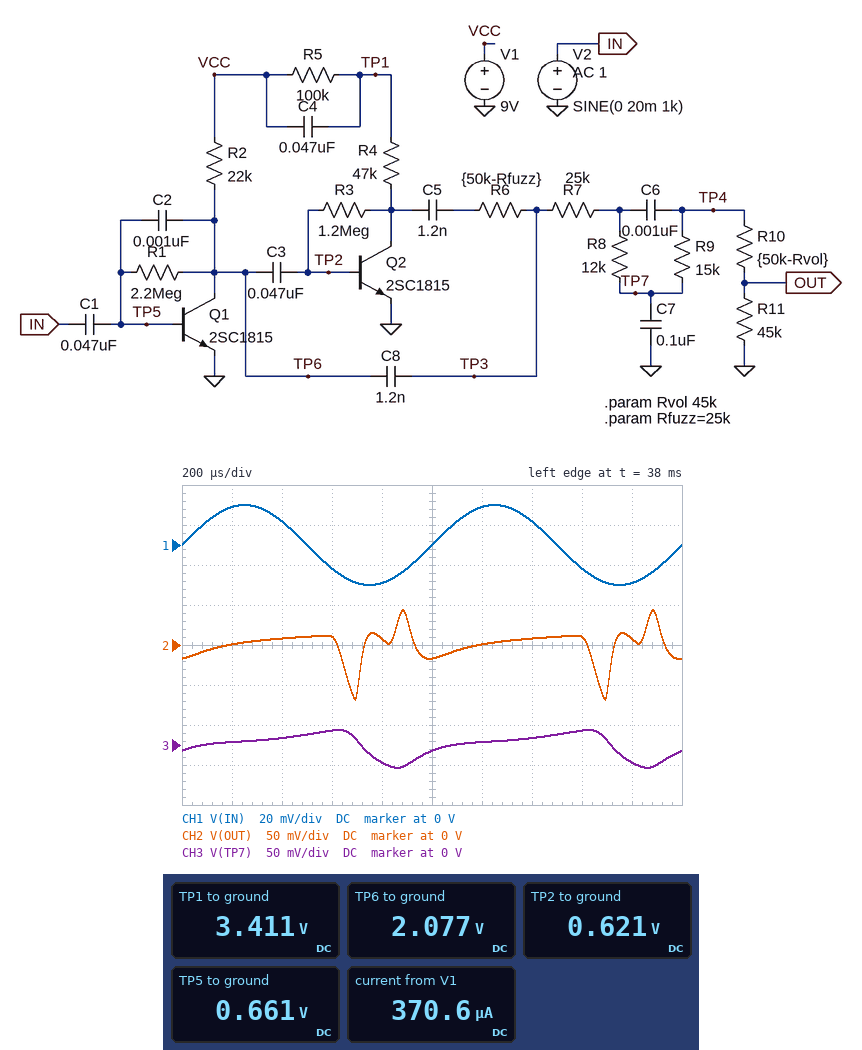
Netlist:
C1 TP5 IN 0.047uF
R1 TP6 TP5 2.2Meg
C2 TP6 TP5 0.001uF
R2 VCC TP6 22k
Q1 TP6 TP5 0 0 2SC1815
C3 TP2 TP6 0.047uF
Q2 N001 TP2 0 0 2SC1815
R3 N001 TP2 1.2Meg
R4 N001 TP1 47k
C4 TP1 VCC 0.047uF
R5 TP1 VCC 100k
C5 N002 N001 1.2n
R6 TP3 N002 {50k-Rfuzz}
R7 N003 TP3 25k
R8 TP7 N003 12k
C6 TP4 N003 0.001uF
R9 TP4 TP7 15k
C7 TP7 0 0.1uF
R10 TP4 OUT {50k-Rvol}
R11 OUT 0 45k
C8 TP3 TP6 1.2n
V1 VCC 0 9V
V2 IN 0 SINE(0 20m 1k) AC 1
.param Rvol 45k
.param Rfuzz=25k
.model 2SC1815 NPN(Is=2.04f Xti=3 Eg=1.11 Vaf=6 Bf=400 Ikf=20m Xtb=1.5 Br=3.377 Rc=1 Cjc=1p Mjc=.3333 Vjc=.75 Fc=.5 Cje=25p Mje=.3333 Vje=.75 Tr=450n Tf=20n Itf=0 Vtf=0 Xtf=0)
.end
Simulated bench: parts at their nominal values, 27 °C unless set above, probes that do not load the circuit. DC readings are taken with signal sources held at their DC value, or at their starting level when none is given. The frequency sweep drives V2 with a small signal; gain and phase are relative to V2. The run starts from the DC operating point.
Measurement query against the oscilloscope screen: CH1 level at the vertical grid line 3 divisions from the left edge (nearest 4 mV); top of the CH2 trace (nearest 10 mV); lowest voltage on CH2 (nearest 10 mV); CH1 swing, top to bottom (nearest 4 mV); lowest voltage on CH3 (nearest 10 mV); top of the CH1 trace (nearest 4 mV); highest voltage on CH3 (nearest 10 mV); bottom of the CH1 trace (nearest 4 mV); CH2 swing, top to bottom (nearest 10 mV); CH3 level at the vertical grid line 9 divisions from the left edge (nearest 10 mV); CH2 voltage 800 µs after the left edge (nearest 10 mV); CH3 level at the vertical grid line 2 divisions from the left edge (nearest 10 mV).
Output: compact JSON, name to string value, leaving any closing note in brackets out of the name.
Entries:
{"CH1 level at the vertical grid line 3 divisions from the left edge": "-12 mV", "top of the CH2 trace": "40 mV", "lowest voltage on CH2": "-70 mV", "CH1 swing, top to bottom": "40 mV", "lowest voltage on CH3": "-30 mV", "top of the CH1 trace": "20 mV", "highest voltage on CH3": "20 mV", "bottom of the CH1 trace": "-20 mV", "CH2 swing, top to bottom": "110 mV", "CH3 level at the vertical grid line 9 divisions from the left edge": "-20 mV", "CH2 voltage 800 µs after the left edge": "10 mV", "CH3 level at the vertical grid line 2 divisions from the left edge": "10 mV"}
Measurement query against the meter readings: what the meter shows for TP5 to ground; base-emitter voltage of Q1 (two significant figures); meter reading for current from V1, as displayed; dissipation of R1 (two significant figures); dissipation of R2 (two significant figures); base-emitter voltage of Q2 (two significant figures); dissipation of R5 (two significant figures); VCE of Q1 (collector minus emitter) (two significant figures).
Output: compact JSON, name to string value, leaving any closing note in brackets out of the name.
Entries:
{"what the meter shows for TP5 to ground": "0.661 V", "base-emitter voltage of Q1": "660 mV", "meter reading for current from V1, as displayed": "370.6 µA", "dissipation of R1": "910 nW", "dissipation of R2": "2.2 mW", "base-emitter voltage of Q2": "620 mV", "dissipation of R5": "310 µW", "VCE of Q1 (collector minus emitter)": "2.1 V"}
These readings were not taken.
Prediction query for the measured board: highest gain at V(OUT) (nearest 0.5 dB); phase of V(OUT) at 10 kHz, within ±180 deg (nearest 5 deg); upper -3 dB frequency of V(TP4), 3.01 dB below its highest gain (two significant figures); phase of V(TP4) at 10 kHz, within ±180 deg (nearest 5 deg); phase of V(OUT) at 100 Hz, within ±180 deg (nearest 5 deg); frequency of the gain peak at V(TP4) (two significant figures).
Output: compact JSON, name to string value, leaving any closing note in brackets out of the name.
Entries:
{"highest gain at V(OUT)": "25.5 dB", "phase of V(OUT) at 10 kHz, within ±180 deg": "-45 deg", "upper -3 dB frequency of V(TP4), 3.01 dB below its highest gain": "11 kHz", "phase of V(TP4) at 10 kHz, within ±180 deg": "-45 deg", "phase of V(OUT) at 100 Hz, within ±180 deg": "110 deg", "frequency of the gain peak at V(TP4)": "4.1 kHz"}
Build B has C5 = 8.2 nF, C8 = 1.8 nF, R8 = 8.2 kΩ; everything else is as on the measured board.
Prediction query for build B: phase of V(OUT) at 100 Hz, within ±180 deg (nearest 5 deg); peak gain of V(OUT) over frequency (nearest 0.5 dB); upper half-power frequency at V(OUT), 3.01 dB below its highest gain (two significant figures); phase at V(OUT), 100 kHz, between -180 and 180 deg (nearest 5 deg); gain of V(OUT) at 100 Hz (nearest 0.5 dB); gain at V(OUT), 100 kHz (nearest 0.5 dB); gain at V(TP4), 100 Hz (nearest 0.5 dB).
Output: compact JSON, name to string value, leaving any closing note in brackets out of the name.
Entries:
{"phase of V(OUT) at 100 Hz, within ±180 deg": "90 deg", "peak gain of V(OUT) over frequency": "37.5 dB", "upper half-power frequency at V(OUT), 3.01 dB below its highest gain": "420 Hz", "phase at V(OUT), 100 kHz, between -180 and 180 deg": "-155 deg", "gain of V(OUT) at 100 Hz": "33.0 dB", "gain at V(OUT), 100 kHz": "3.0 dB", "gain at V(TP4), 100 Hz": "34.0 dB"}
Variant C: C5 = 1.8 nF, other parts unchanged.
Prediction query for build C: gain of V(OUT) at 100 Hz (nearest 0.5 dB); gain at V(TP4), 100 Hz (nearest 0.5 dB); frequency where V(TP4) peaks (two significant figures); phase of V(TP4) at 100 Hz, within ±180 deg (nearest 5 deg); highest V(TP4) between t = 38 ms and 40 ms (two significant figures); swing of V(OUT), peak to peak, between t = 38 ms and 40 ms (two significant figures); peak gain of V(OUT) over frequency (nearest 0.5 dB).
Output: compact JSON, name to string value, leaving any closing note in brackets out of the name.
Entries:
{"gain of V(OUT) at 100 Hz": "20.5 dB", "gain at V(TP4), 100 Hz": "21.5 dB", "frequency where V(TP4) peaks": "330 Hz", "phase of V(TP4) at 100 Hz, within ±180 deg": "105 deg", "highest V(TP4) between t = 38 ms and 40 ms": "52 mV", "swing of V(OUT), peak to peak, between t = 38 ms and 40 ms": "120 mV", "peak gain of V(OUT) over frequency": "26.5 dB"}
